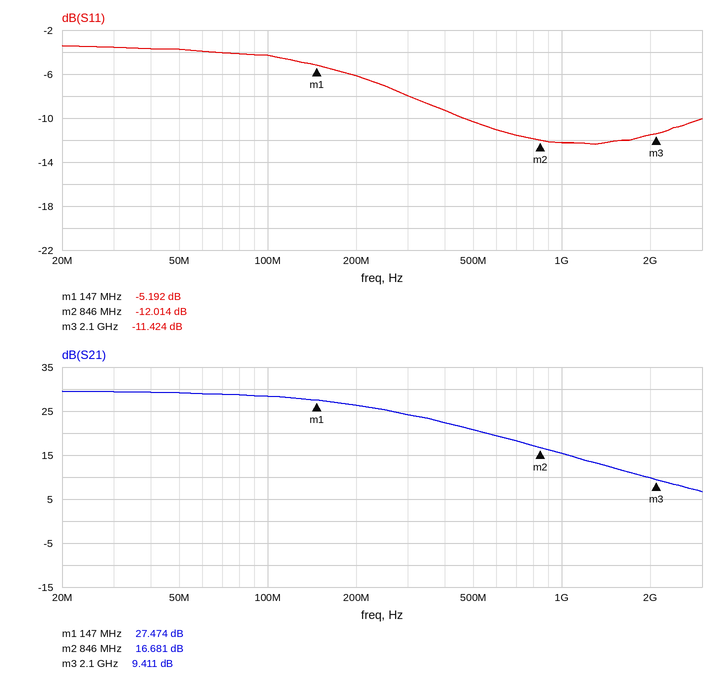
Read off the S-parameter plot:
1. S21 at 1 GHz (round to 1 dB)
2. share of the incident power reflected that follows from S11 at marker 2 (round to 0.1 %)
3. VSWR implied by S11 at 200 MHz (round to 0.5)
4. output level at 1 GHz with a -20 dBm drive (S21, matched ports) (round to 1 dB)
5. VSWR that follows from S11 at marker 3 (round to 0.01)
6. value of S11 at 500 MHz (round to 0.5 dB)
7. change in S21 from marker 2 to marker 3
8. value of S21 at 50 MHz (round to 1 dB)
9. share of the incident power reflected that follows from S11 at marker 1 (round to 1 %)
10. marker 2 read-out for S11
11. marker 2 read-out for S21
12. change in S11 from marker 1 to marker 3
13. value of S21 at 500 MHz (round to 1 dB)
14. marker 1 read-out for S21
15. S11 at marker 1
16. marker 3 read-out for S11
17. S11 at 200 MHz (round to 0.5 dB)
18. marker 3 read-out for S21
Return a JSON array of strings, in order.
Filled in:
["15 dB", "6.3 %", "3.0", "-5 dBm", "1.73", "-10.5 dB", "-7.270 dB", "29 dB", "30 %", "-12.014 dB", "16.681 dB", "-6.232 dB", "21 dB", "27.474 dB", "-5.192 dB", "-11.424 dB", "-6.0 dB", "9.411 dB"]
